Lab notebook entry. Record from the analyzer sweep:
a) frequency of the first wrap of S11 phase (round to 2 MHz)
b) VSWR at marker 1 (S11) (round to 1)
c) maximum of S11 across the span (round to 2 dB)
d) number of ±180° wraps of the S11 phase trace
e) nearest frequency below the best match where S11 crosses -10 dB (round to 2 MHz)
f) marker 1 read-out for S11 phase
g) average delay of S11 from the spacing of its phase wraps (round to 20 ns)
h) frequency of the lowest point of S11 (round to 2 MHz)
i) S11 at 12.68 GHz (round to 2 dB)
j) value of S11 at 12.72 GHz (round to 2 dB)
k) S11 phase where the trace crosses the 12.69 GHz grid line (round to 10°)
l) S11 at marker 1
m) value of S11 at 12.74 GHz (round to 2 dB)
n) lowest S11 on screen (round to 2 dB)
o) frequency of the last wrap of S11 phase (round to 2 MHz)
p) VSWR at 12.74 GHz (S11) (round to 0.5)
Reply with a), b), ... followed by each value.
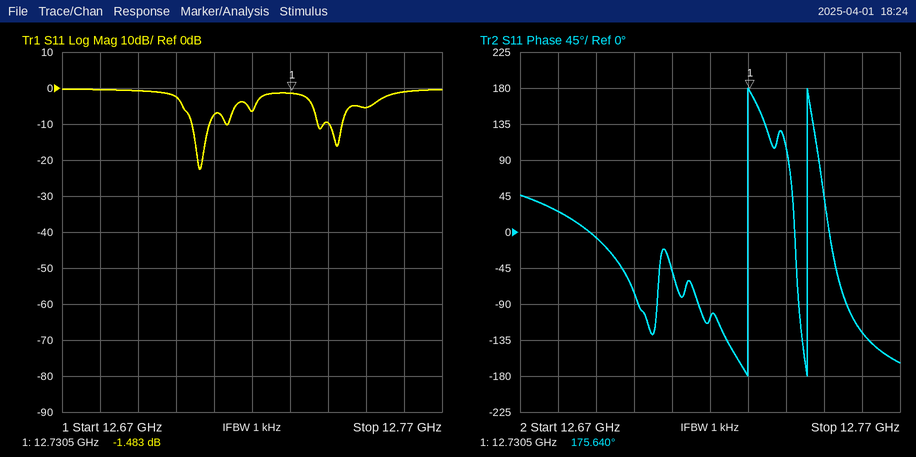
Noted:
a) 12.730 GHz
b) 12
c) 0 dB
d) 2
e) 12.704 GHz
f) 175.640°
g) 60 ns
h) 12.706 GHz
i) 0 dB
j) -6 dB
k) -10°
l) -1.483 dB
m) -10 dB
n) -22 dB
o) 12.746 GHz
p) 2.0
